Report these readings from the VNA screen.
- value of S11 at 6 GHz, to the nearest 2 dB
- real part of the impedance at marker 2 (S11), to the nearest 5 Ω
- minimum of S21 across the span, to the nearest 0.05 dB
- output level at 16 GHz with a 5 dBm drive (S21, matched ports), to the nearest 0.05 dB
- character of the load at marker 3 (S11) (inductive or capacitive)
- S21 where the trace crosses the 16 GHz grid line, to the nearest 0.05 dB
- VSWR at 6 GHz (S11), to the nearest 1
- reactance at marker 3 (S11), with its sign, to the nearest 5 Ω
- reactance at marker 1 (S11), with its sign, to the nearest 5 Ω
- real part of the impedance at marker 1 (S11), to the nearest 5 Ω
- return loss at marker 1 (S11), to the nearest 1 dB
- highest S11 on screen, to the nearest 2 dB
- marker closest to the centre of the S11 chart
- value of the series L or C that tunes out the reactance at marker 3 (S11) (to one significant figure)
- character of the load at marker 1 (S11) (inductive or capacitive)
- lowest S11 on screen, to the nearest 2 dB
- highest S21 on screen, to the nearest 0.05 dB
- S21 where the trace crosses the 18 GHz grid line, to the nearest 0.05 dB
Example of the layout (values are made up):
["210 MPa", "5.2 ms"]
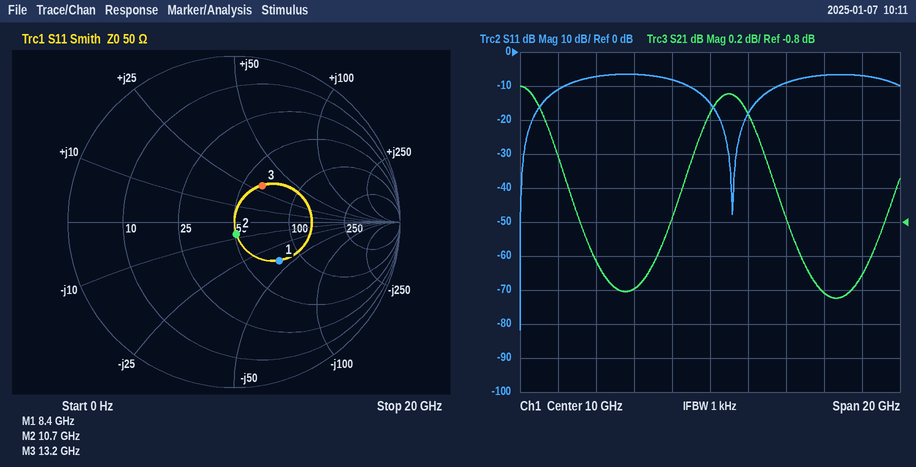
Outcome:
["-6 dB", "50 Ω", "-1.25 dB", "3.80 dBm", "inductive", "-1.20 dB", "3", "+30 Ω", "-40 Ω", "75 Ω", "9 dB", "-6 dB", "marker 2", "400 fF", "capacitive", "-82 dB", "0.00 dB", "-1.10 dB"]
